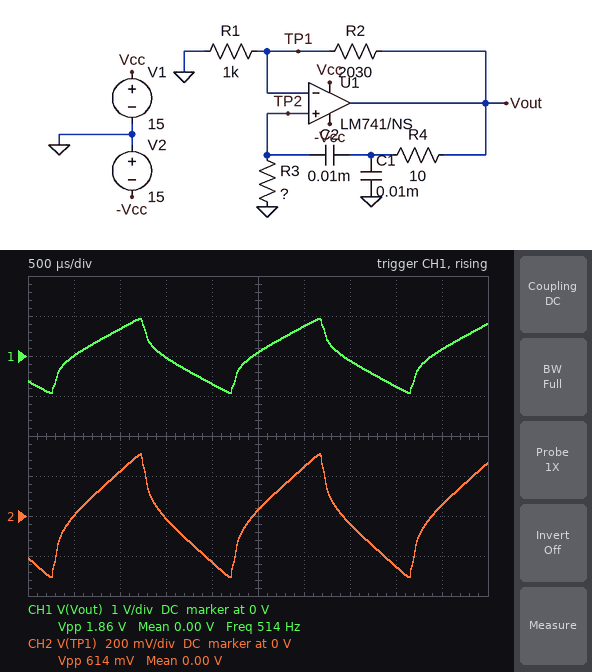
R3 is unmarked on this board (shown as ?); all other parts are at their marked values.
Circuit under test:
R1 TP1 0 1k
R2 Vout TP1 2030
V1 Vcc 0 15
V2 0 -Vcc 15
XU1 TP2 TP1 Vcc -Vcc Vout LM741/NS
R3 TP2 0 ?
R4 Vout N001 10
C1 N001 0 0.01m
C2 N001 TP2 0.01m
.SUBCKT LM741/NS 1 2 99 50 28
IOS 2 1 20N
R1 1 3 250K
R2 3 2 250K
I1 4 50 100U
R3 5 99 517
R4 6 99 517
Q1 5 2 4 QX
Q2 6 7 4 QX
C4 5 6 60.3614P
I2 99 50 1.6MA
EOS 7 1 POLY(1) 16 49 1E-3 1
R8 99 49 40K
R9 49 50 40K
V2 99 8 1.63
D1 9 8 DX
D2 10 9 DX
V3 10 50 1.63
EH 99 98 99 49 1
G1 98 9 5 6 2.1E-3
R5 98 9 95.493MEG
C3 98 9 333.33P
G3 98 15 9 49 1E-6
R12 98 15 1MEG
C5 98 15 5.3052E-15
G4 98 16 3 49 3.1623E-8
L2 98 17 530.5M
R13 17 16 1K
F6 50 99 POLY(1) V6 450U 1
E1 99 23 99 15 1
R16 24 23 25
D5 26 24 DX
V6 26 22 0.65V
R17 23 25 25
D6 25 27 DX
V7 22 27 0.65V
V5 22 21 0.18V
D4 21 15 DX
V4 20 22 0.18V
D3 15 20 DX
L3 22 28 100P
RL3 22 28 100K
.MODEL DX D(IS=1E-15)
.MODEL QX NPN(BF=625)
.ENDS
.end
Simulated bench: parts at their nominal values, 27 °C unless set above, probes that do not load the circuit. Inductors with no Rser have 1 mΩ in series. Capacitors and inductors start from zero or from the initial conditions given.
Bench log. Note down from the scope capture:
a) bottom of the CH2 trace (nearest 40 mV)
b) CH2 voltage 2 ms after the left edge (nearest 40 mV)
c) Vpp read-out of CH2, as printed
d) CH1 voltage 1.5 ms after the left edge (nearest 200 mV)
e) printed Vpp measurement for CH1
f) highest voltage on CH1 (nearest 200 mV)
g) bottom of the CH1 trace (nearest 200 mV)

-320 mV
-240 mV
614 mV
0 V
1.86 V
1.0 V
-1.0 V
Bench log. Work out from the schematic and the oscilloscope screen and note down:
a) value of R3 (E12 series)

22 Ω
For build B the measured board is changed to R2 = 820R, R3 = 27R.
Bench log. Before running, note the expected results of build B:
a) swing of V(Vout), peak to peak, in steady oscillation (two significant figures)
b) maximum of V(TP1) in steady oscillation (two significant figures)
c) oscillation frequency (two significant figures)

1.3 V
360 mV
850 Hz
